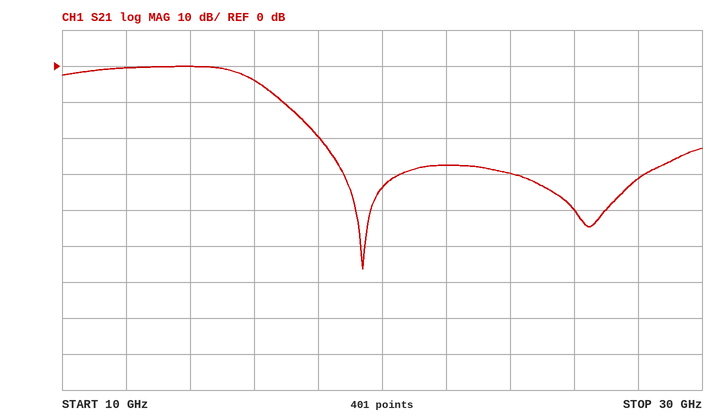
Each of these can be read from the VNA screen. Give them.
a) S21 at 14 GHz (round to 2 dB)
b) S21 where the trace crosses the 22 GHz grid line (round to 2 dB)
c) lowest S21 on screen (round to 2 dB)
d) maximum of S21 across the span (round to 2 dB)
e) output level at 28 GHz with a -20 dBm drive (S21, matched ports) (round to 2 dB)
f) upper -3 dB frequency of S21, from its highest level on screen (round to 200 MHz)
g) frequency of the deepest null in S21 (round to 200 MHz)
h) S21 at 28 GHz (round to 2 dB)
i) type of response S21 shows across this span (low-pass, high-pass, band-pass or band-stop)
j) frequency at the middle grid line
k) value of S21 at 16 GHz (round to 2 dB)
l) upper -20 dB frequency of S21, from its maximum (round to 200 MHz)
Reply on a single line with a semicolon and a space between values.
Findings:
0 dB; -28 dB; -56 dB; 0 dB; -52 dBm; 15.8 GHz; 19.4 GHz; -32 dB; low-pass; 20 GHz; -4 dB; 18.0 GHz
